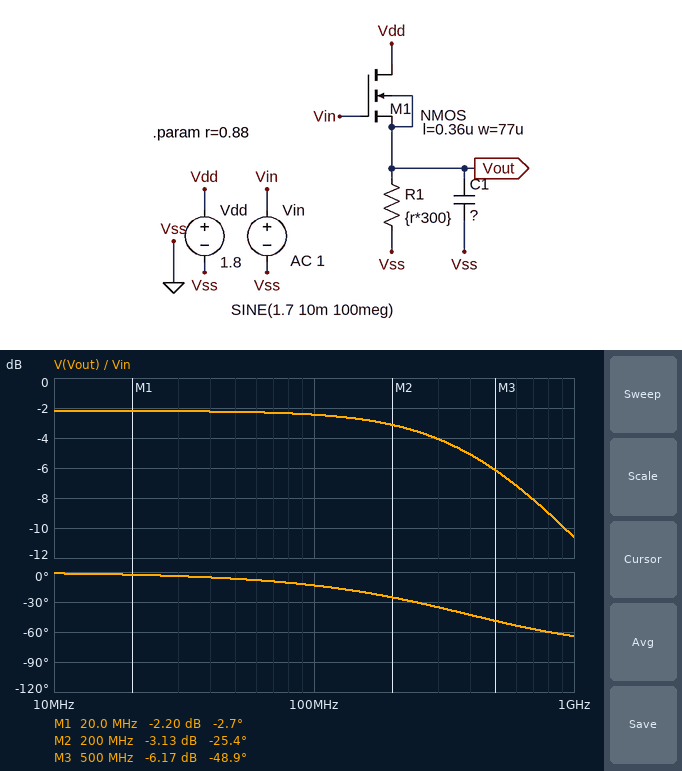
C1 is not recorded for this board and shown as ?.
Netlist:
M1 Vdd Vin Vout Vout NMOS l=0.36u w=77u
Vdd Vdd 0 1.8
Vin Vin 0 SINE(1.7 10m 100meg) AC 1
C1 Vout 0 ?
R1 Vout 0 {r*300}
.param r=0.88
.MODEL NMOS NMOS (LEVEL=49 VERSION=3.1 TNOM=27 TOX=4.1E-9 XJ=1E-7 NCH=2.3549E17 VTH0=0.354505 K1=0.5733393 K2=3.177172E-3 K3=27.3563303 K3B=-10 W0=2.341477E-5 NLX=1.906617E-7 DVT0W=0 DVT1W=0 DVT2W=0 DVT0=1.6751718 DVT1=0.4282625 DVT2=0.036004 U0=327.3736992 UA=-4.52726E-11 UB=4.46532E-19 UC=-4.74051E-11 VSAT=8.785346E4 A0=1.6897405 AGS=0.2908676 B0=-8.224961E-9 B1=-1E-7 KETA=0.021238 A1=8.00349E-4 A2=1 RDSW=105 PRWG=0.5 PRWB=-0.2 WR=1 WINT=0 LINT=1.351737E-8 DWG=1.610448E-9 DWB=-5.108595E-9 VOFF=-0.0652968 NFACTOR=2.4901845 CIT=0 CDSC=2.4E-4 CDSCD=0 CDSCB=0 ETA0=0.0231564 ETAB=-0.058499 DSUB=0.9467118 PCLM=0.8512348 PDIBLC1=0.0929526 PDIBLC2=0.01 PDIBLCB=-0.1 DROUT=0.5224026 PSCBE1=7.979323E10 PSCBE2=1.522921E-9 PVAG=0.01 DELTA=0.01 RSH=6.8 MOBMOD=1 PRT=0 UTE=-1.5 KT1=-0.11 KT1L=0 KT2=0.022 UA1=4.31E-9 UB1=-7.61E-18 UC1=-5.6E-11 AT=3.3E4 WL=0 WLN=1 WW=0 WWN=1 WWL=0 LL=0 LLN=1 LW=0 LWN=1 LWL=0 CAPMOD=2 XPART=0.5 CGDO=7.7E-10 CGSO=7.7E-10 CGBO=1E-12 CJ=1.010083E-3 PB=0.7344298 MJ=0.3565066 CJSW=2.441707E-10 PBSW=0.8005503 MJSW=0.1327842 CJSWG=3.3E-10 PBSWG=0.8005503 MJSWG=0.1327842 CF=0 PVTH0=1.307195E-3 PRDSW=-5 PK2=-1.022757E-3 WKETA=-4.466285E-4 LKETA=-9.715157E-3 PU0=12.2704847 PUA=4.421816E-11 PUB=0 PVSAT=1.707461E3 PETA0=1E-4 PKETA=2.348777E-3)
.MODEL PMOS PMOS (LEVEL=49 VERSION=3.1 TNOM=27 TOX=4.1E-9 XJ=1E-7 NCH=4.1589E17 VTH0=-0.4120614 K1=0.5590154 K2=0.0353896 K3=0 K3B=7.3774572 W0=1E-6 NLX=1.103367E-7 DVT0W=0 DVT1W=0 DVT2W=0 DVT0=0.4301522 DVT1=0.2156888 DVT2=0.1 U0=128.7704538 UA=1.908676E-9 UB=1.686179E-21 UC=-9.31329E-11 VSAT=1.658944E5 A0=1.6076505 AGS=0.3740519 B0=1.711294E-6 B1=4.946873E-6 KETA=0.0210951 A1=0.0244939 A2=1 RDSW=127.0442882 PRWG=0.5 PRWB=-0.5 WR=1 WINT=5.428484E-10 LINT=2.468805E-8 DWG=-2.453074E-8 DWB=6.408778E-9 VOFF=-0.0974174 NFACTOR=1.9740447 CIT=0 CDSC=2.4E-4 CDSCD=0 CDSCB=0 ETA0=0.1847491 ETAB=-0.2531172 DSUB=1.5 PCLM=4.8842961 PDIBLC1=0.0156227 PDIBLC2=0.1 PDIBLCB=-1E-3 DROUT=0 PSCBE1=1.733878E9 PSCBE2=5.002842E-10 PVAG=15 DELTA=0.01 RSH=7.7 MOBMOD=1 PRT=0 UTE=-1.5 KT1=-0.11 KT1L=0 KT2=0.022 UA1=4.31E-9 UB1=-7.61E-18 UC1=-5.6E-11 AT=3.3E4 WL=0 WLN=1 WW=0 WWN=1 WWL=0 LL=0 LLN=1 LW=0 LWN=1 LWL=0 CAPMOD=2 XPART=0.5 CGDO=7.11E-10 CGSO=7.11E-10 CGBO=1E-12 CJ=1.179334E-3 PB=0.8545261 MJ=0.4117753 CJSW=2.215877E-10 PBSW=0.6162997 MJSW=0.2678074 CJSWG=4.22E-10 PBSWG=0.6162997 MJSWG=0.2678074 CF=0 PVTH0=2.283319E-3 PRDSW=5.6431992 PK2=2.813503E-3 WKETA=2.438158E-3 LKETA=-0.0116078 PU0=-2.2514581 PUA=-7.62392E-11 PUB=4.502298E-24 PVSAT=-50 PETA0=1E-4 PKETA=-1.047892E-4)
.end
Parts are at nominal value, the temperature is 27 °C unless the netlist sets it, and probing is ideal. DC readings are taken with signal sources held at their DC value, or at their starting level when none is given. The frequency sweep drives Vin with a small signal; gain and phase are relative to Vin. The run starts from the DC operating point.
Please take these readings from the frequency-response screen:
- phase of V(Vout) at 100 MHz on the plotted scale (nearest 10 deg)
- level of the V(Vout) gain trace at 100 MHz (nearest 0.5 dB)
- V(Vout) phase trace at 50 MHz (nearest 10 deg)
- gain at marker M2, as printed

-10 deg
-2.5 dB
-10 deg
-3.13 dB
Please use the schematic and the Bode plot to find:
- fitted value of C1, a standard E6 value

6.8 pF
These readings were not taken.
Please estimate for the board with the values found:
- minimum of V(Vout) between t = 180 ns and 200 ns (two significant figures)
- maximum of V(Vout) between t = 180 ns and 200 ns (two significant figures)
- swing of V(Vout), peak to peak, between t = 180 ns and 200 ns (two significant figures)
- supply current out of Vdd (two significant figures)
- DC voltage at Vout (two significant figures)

830 mV
850 mV
15 mV
3.2 mA
840 mV
